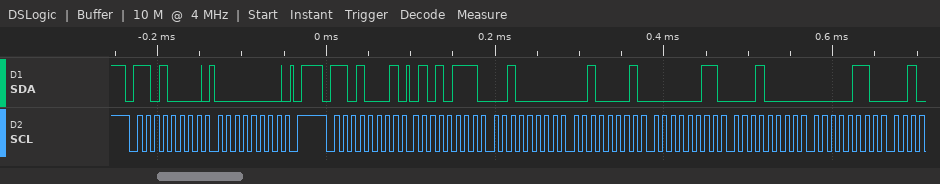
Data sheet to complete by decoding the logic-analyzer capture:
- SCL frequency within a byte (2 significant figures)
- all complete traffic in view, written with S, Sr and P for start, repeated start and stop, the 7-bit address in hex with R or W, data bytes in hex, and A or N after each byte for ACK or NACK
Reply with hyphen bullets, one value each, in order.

- 100 kHz
- S 68W A 00 A P S 68R A 57 A 20 A 21 A 03 A 10 A 06 A
